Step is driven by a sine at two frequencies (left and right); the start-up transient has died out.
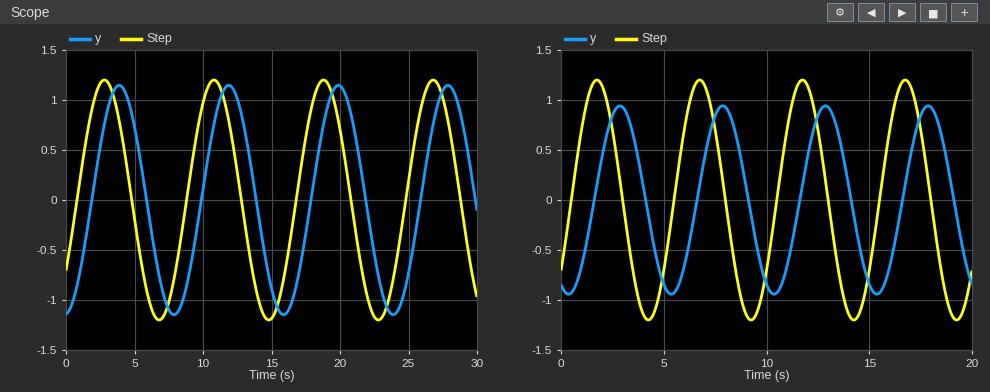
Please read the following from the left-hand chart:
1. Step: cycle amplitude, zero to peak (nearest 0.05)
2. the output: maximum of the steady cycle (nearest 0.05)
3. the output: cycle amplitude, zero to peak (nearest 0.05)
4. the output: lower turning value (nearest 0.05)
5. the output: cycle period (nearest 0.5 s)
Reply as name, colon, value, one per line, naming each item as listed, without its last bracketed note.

Step: cycle amplitude, zero to peak: 1.20
the output: maximum of the steady cycle: 1.15
the output: cycle amplitude, zero to peak: 1.15
the output: lower turning value: -1.15
the output: cycle period: 8.0 s
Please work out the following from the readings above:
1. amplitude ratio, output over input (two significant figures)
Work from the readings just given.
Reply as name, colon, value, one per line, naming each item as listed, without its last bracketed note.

amplitude ratio, output over input: 0.96
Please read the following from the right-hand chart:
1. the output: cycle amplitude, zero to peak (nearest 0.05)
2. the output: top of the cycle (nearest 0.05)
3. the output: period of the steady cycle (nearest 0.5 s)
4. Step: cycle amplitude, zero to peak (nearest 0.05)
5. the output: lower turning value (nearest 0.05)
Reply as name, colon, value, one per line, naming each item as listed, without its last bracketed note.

the output: cycle amplitude, zero to peak: 0.95
the output: top of the cycle: 0.95
the output: period of the steady cycle: 5.0 s
Step: cycle amplitude, zero to peak: 1.20
the output: lower turning value: -0.95
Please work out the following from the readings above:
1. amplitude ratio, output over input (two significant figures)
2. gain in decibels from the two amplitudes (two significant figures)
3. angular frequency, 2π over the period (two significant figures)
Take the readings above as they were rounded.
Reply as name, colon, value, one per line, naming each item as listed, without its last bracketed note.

amplitude ratio, output over input: 0.79
gain in decibels from the two amplitudes: -2.0 dB
angular frequency, 2π over the period: 1.3 rad/s
